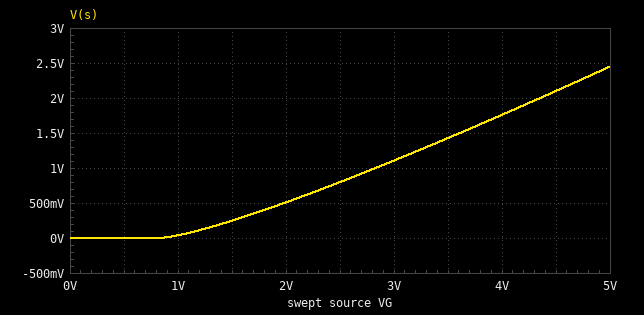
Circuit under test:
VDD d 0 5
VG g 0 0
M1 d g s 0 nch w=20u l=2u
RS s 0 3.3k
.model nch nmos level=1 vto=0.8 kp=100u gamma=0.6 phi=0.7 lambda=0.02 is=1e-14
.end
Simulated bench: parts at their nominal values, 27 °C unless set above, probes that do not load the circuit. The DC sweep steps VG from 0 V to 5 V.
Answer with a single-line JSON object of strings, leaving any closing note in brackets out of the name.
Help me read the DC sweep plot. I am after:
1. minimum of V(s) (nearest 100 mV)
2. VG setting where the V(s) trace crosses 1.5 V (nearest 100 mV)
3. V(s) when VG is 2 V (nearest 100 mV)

{"minimum of V(s)": "0 V", "VG setting where the V(s) trace crosses 1.5 V": "3.6 V", "V(s) when VG is 2 V": "500 mV"}
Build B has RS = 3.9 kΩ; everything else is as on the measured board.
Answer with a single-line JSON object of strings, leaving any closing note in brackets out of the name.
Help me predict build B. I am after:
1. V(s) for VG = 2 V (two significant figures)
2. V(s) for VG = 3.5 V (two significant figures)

{"V(s) for VG = 2 V": "530 mV", "V(s) for VG = 3.5 V": "1.5 V"}
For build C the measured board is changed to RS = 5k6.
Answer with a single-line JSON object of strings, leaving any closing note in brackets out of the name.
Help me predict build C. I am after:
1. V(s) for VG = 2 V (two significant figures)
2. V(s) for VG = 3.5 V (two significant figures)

{"V(s) for VG = 2 V": "580 mV", "V(s) for VG = 3.5 V": "1.6 V"}
